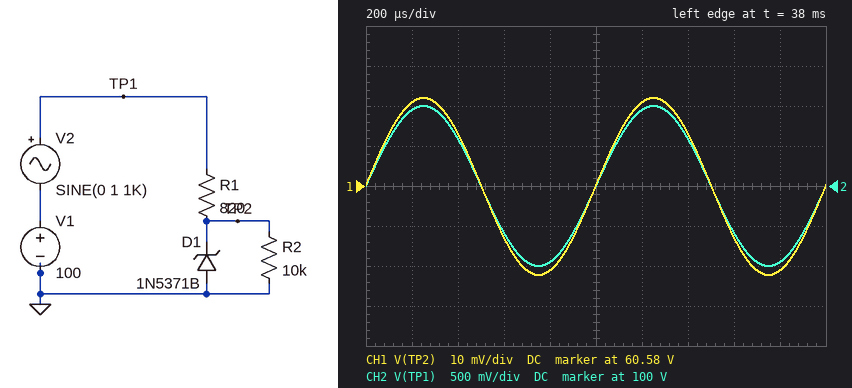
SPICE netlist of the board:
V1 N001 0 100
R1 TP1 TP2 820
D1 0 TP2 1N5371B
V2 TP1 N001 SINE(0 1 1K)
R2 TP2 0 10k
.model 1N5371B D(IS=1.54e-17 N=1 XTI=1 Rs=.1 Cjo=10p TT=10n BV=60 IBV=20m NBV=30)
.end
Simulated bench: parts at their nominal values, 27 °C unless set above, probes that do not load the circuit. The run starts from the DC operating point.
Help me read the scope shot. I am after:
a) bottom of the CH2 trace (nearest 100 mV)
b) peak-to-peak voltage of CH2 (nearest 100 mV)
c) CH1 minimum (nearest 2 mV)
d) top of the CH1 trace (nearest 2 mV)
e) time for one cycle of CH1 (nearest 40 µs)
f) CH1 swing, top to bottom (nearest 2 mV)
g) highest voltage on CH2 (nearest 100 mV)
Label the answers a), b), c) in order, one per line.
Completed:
a) 99.0 V
b) 2.0 V
c) 60.558 V
d) 60.602 V
e) 1.00 ms
f) 44 mV
g) 101.0 V
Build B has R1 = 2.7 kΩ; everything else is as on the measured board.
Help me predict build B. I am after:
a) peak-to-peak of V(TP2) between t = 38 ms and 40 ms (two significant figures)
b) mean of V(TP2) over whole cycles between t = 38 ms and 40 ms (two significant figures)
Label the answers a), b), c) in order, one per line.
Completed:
a) 61 mV
b) 59 V
